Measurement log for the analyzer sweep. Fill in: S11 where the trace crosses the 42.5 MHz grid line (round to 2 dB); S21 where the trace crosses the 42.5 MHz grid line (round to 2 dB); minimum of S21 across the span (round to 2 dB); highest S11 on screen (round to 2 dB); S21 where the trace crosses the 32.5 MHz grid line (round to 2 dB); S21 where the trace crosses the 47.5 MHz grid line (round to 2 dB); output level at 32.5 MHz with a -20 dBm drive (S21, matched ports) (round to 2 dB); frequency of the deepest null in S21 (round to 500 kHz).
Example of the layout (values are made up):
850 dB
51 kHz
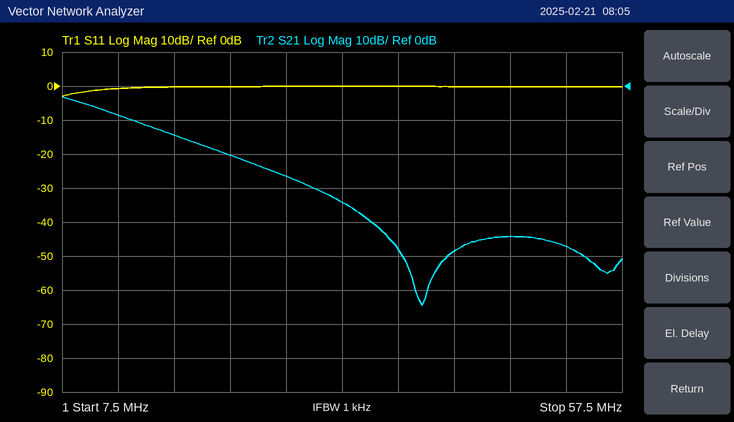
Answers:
0 dB
-48 dB
-64 dB
0 dB
-34 dB
-44 dB
-54 dBm
39.5 MHz
